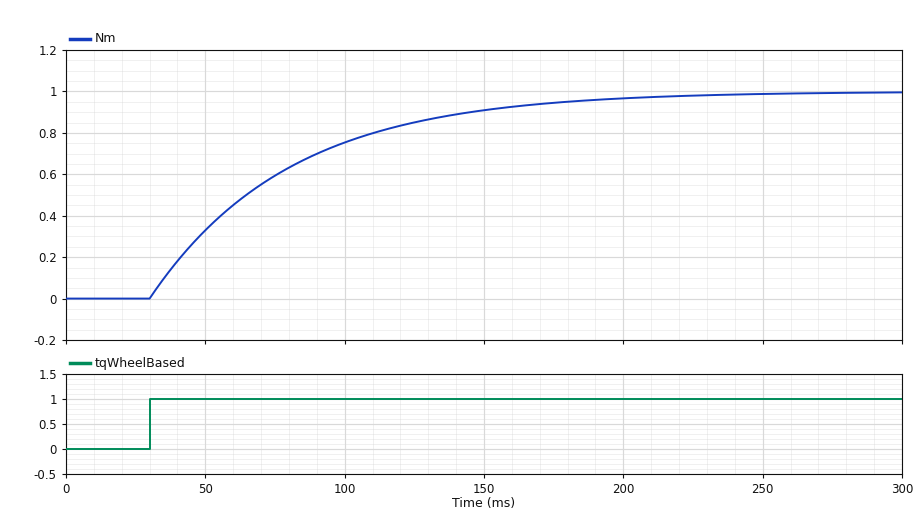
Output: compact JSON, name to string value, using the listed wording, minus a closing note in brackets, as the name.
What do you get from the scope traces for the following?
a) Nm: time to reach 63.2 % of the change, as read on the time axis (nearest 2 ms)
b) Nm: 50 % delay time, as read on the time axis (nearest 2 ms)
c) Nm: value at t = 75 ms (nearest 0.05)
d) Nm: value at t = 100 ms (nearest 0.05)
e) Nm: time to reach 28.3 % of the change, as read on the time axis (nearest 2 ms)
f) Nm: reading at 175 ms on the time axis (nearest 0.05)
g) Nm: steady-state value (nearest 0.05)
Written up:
{"Nm: time to reach 63.2 % of the change, as read on the time axis": "80 ms", "Nm: 50 % delay time, as read on the time axis": "64 ms", "Nm: value at t = 75 ms": "0.60", "Nm: value at t = 100 ms": "0.75", "Nm: time to reach 28.3 % of the change, as read on the time axis": "46 ms", "Nm: reading at 175 ms on the time axis": "0.95", "Nm: steady-state value": "1.00"}
